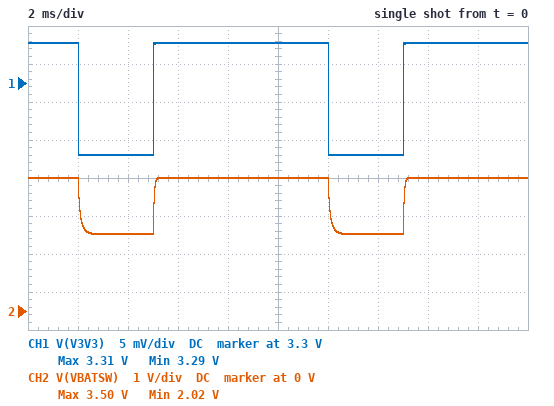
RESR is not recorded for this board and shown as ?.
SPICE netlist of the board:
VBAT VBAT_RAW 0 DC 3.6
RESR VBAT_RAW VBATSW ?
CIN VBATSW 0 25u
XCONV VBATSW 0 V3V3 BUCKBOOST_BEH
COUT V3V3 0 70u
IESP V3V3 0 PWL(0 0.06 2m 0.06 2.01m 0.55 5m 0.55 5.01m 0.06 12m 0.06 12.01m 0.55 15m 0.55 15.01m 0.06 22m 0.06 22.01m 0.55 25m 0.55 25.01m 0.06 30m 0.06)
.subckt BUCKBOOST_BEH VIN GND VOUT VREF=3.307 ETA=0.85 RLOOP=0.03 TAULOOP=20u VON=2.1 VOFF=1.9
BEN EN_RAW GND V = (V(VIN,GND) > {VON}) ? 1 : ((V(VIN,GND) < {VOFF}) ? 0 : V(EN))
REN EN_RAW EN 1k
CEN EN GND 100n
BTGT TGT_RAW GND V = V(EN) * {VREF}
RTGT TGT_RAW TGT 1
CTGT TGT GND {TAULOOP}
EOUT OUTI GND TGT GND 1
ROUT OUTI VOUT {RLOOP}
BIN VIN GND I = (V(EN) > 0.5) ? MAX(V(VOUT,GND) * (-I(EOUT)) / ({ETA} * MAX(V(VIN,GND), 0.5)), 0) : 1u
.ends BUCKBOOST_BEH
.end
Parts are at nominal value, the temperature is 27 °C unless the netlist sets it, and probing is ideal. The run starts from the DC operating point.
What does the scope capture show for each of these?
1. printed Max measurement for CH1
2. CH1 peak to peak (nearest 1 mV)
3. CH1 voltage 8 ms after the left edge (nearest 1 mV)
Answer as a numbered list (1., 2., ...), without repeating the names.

1. 3.31 V
2. 15 mV
3. 3.305 V
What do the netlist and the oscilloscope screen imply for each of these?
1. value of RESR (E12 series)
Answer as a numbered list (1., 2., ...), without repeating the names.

1. 1.5 Ω
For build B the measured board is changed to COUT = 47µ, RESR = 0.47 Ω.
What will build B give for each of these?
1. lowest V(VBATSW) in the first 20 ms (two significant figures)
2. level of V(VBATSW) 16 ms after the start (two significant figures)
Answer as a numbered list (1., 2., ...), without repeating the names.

1. 3.3 V
2. 3.6 V
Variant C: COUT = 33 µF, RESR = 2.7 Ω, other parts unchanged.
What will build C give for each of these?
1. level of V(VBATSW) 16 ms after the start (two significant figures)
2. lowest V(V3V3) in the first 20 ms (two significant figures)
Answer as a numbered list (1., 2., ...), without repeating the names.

1. 3.4 V
2. 1.8 V
